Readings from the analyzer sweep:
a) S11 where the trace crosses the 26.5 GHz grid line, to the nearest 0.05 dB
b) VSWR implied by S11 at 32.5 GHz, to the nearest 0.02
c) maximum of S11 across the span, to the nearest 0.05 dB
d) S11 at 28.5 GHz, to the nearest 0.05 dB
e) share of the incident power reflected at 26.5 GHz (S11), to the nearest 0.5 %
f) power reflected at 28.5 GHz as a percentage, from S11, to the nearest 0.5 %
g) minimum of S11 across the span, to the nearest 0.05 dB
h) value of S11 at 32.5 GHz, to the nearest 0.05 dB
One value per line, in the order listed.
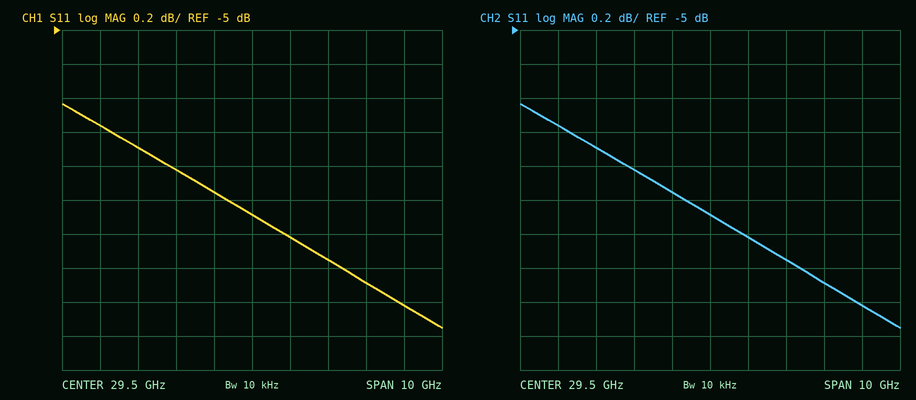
-5.70 dB
2.80
-5.45 dB
-5.95 dB
27.0 %
25.5 %
-6.75 dB
-6.50 dB
